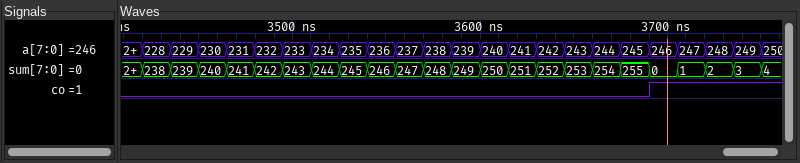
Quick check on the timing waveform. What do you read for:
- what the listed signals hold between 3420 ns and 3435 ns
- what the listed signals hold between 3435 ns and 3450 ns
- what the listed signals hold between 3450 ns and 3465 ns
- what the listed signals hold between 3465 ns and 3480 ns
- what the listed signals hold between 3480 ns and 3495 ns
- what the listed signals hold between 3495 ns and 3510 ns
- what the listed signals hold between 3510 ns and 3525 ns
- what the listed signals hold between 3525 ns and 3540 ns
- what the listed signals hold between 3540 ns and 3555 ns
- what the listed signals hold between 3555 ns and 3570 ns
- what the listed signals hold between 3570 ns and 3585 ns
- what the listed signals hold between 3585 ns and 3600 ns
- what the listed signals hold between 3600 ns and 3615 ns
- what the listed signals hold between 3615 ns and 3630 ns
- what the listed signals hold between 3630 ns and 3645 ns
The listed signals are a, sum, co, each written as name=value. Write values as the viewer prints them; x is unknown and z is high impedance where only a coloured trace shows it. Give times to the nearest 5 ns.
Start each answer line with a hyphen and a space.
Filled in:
- a=228, sum=238, co=0
- a=229, sum=239, co=0
- a=230, sum=240, co=0
- a=231, sum=241, co=0
- a=232, sum=242, co=0
- a=233, sum=243, co=0
- a=234, sum=244, co=0
- a=235, sum=245, co=0
- a=236, sum=246, co=0
- a=237, sum=247, co=0
- a=238, sum=248, co=0
- a=239, sum=249, co=0
- a=240, sum=250, co=0
- a=241, sum=251, co=0
- a=242, sum=252, co=0
